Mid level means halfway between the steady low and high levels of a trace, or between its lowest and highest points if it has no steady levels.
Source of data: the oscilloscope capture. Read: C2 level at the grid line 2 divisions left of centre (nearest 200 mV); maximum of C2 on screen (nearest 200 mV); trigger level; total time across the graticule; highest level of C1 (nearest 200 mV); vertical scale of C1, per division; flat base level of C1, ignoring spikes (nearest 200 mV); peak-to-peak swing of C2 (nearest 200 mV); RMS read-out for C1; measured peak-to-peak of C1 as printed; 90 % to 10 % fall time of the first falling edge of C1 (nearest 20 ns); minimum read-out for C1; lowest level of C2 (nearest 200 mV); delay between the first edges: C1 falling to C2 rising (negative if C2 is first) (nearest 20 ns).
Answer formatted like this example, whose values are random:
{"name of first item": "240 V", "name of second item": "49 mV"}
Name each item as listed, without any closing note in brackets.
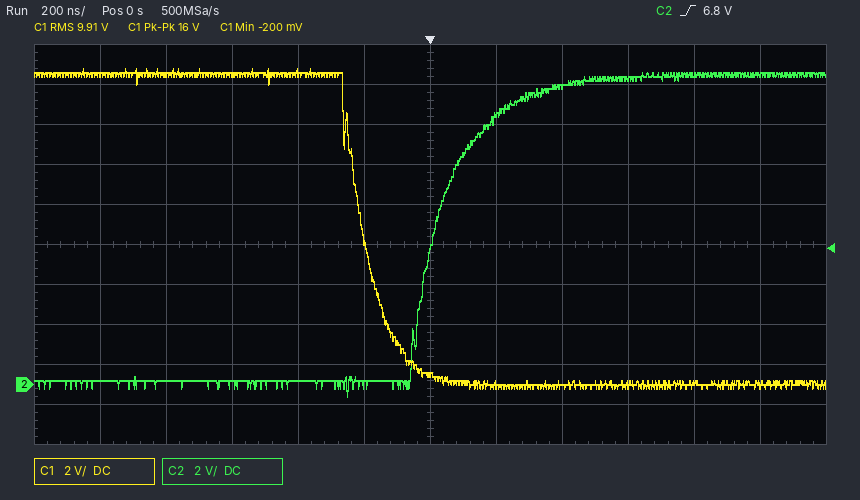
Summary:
{"C2 level at the grid line 2 divisions left of centre": "200 mV", "maximum of C2 on screen": "15.6 V", "trigger level": "6.8 V", "total time across the graticule": "2.4 µs", "highest level of C1": "15.8 V", "vertical scale of C1, per division": "2 V", "flat base level of C1, ignoring spikes": "0.0 V", "peak-to-peak swing of C2": "16.2 V", "RMS read-out for C1": "9.91 V", "measured peak-to-peak of C1 as printed": "16 V", "90 % to 10 % fall time of the first falling edge of C1": "180 ns", "minimum read-out for C1": "-200 mV", "lowest level of C2": "-600 mV", "delay between the first edges: C1 falling to C2 rising (negative if C2 is first)": "+220 ns"}
